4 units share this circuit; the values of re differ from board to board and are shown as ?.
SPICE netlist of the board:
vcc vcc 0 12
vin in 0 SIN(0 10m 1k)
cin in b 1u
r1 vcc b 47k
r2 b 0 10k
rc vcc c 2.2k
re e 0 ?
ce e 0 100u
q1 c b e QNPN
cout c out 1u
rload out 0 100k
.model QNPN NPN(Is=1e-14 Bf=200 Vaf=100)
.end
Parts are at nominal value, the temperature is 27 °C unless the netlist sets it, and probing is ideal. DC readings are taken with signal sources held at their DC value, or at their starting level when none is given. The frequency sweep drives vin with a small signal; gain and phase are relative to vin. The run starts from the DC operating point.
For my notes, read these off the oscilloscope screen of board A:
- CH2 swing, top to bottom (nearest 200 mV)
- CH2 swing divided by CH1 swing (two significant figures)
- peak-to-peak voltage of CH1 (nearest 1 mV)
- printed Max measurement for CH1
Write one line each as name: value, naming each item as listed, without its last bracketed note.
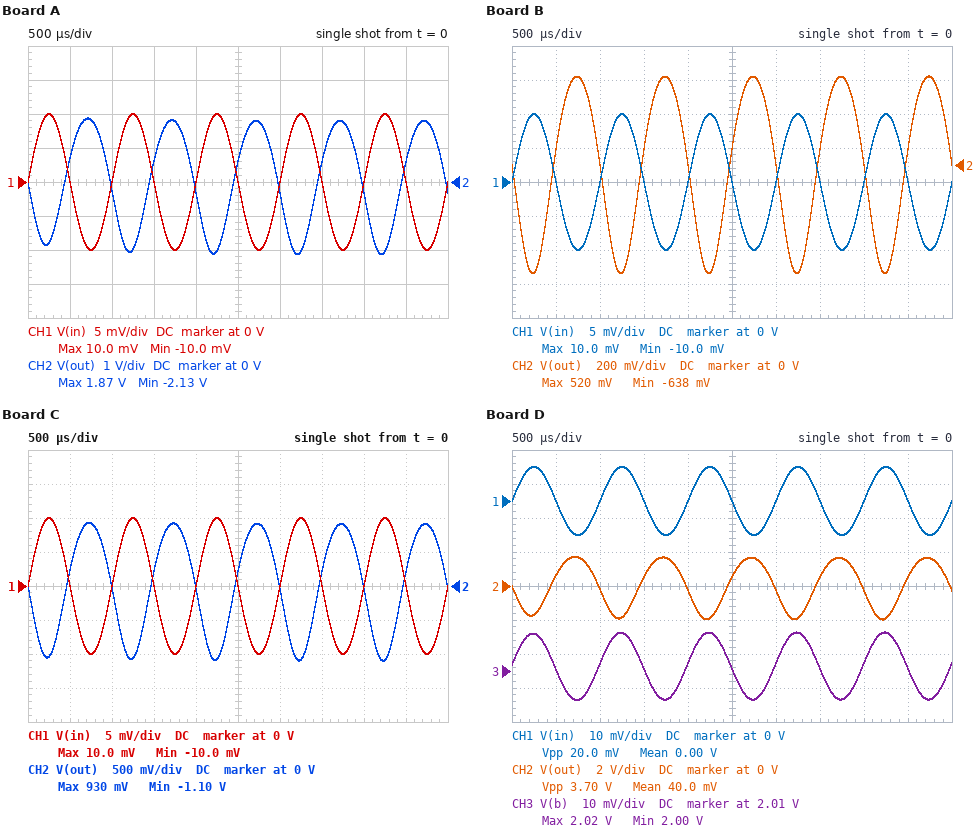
CH2 swing, top to bottom: 4.0 V
CH2 swing divided by CH1 swing: 200
peak-to-peak voltage of CH1: 20 mV
printed Max measurement for CH1: 10.0 mV
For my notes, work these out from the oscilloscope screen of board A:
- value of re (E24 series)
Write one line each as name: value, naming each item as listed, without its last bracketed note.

value of re: 510 Ω
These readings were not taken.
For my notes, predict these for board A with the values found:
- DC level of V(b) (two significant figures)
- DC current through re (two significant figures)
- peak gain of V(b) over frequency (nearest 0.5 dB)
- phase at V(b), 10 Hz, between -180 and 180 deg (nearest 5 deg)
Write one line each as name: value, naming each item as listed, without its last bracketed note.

DC level of V(b): 2.0 V
DC current through re: 2.6 mA
peak gain of V(b) over frequency: 0 dB
phase at V(b), 10 Hz, between -180 and 180 deg: 55 deg
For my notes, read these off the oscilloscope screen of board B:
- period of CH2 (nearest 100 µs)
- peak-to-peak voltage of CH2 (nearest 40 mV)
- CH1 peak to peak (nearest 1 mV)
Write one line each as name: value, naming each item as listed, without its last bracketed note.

period of CH2: 1.0 ms
peak-to-peak voltage of CH2: 1.16 V
CH1 peak to peak: 20 mV
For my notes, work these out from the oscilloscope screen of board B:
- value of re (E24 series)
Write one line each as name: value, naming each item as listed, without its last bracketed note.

value of re: 2 kΩ
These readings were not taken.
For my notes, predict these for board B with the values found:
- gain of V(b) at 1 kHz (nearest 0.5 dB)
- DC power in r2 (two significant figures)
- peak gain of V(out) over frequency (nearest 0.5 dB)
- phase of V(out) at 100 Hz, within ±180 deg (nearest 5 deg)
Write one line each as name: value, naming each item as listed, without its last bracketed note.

gain of V(b) at 1 kHz: 0 dB
DC power in r2: 430 µW
peak gain of V(out) over frequency: 35.5 dB
phase of V(out) at 100 Hz, within ±180 deg: -135 deg
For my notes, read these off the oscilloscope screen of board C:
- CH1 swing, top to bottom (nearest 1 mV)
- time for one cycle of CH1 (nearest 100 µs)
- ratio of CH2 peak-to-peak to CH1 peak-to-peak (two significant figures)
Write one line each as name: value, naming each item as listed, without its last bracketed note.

CH1 swing, top to bottom: 20 mV
time for one cycle of CH1: 1.0 ms
ratio of CH2 peak-to-peak to CH1 peak-to-peak: 100
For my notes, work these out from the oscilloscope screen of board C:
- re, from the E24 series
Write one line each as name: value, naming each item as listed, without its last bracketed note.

re, from the E24 series: 1.1 kΩ
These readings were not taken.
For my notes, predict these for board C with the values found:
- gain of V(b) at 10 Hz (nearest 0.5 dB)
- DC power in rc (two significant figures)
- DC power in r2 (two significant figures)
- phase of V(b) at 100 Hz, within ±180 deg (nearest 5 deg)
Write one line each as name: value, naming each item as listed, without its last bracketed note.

gain of V(b) at 10 Hz: -8.0 dB
DC power in rc: 3.5 mW
DC power in r2: 420 µW
phase of V(b) at 100 Hz, within ±180 deg: 20 deg
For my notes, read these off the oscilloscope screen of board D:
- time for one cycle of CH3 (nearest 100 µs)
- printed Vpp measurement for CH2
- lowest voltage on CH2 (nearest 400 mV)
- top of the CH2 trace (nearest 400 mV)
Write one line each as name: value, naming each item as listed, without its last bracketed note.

time for one cycle of CH3: 1.0 ms
printed Vpp measurement for CH2: 3.70 V
lowest voltage on CH2: -2.0 V
top of the CH2 trace: 1.6 V
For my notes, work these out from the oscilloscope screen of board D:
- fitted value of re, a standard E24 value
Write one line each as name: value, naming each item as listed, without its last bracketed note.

fitted value of re, a standard E24 value: 560 Ω
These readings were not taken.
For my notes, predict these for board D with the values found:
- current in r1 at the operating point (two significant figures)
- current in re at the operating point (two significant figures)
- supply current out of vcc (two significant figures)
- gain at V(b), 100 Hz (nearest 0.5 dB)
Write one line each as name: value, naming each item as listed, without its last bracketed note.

current in r1 at the operating point: 210 µA
current in re at the operating point: 2.4 mA
supply current out of vcc: 2.6 mA
gain at V(b), 100 Hz: -3.0 dB
